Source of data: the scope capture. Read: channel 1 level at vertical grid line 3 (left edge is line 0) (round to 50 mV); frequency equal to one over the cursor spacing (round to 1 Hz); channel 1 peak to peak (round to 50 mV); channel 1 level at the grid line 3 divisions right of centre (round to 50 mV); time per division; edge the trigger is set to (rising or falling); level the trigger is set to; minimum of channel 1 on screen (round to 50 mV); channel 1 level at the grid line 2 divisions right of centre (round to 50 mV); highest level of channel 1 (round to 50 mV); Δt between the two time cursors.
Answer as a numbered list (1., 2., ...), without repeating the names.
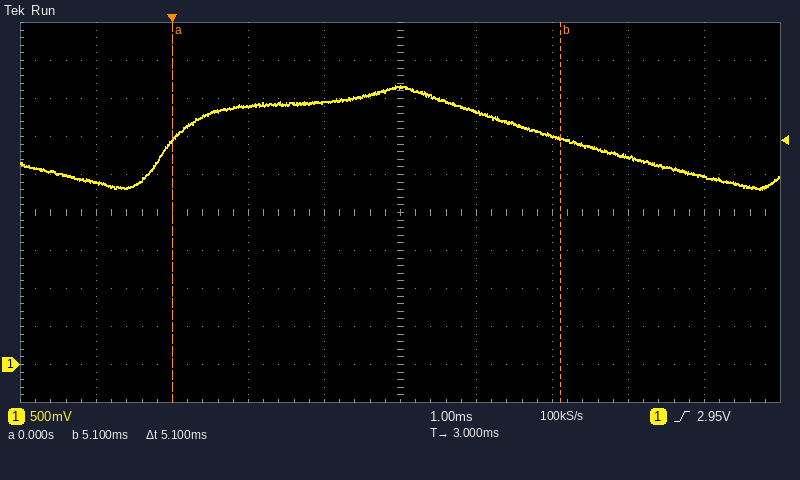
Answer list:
1. 3.40 V
2. 196 Hz
3. 1.35 V
4. 2.75 V
5. 1 ms
6. rising
7. 2.95 V
8. 2.30 V
9. 3.00 V
10. 3.65 V
11. 5.1 ms
